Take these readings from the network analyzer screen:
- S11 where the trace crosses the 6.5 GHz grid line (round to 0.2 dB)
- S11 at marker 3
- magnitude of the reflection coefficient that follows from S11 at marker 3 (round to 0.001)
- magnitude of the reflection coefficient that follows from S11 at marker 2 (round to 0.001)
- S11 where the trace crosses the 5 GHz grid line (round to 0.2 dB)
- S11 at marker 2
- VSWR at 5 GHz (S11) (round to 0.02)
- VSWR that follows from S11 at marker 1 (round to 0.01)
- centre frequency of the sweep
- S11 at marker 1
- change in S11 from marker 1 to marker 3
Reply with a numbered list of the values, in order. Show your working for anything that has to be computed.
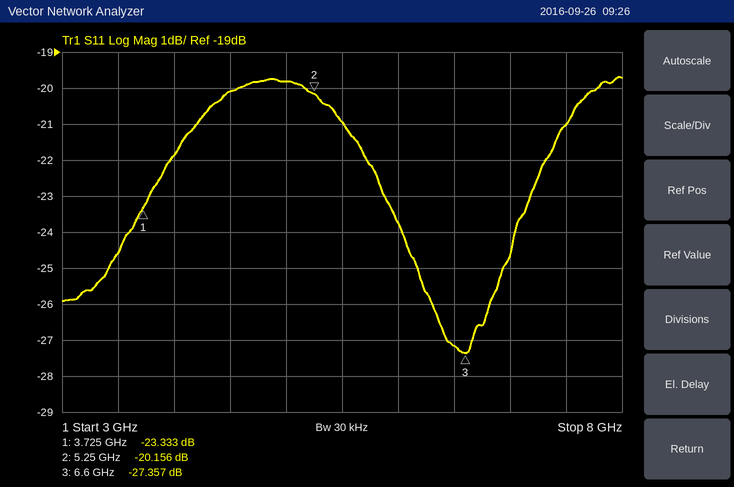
1. -27.2 dB
2. -27.357 dB
3. 10^(-27.357/20) ≈ 0.043
4. 10^(-20.156/20) ≈ 0.098
5. -19.8 dB
6. -20.156 dB
7. |Γ| = 10^(-19.8/20) = 0.1023; VSWR = (1 + 0.1023)/(1 − 0.1023) ≈ 1.23, so 1.22 to the nearest 0.02
8. (1 + 0.0681)/(1 − 0.0681) ≈ 1.15
9. 5.5 GHz
10. -23.333 dB
11. -27.357 − (-23.333) = -4.024 dB
